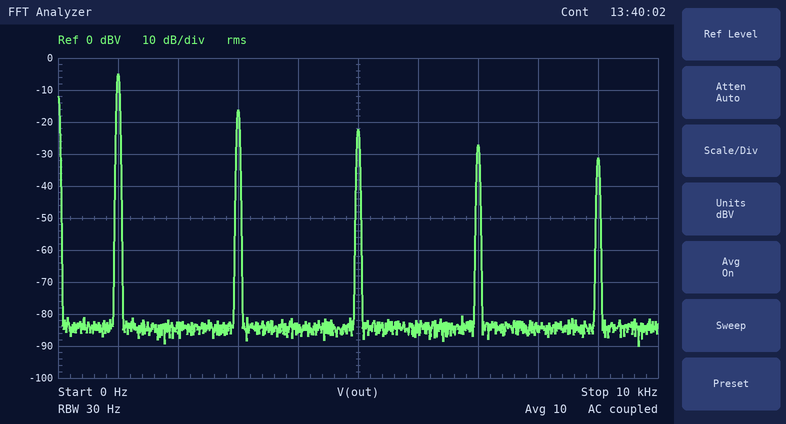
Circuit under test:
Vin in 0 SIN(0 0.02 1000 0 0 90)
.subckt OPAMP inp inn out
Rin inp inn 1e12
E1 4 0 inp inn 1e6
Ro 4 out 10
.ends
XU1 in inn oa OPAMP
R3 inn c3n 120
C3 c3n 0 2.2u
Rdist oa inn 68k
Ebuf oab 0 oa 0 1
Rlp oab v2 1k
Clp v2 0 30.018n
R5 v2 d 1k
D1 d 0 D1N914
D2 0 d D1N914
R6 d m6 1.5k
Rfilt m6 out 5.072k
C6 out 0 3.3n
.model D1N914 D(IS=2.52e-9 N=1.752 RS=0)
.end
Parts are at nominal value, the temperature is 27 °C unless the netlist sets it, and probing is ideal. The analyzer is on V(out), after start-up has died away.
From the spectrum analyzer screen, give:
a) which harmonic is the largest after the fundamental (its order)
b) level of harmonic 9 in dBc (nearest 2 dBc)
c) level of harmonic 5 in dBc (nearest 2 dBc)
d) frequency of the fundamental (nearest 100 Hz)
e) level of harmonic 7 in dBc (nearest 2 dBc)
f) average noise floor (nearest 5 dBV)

3
-26 dBc
-18 dBc
1.0 kHz
-22 dBc
-85 dBV
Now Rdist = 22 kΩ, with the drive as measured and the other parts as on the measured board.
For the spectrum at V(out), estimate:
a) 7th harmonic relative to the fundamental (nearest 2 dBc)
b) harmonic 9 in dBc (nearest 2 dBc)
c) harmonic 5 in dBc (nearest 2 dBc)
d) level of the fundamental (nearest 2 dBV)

-26 dBc
-32 dBc
-20 dBc
-6 dBV
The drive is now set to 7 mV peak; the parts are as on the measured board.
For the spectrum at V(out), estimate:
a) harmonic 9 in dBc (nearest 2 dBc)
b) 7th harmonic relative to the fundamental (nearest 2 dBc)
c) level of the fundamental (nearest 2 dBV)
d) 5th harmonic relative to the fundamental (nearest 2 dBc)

-32 dBc
-26 dBc
-6 dBV
-20 dBc
